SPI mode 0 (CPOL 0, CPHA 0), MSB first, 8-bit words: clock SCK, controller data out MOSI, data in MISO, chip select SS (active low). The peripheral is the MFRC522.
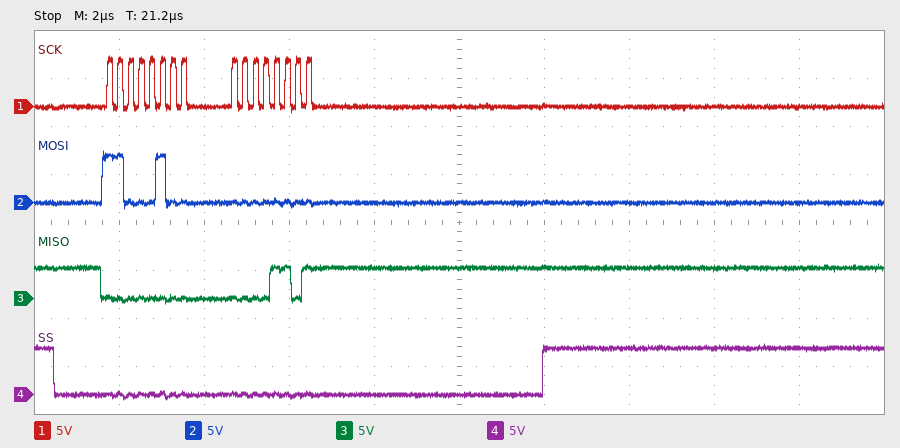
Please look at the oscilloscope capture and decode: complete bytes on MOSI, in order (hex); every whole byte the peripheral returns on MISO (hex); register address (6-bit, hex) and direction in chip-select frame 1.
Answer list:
0xC4 0x00
0x00 0x0D
0x22 read
